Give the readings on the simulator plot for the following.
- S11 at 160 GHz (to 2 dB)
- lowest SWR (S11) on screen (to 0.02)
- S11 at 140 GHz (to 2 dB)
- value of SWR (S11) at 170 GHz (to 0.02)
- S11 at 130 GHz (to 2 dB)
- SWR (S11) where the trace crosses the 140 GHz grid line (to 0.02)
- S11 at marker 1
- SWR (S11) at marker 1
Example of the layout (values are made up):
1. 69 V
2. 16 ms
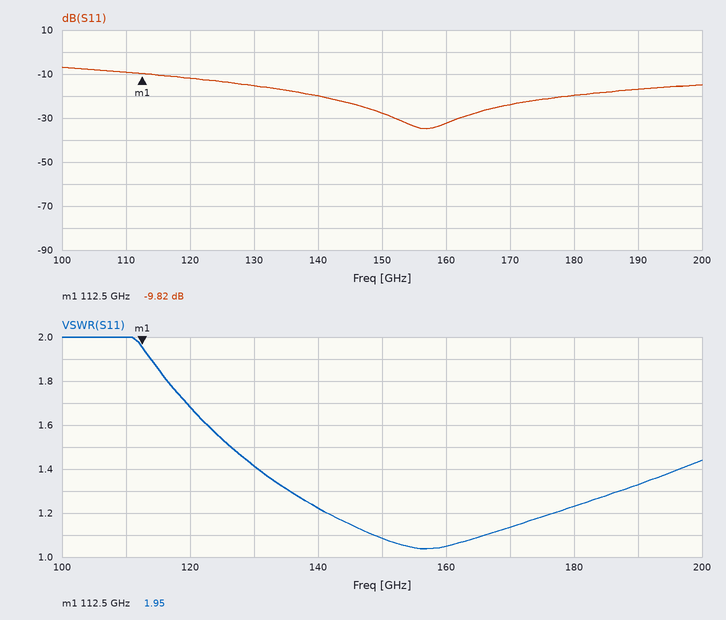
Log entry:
1. -32 dB
2. 1.04
3. -20 dB
4. 1.14
5. -16 dB
6. 1.22
7. -9.82 dB
8. 1.95
